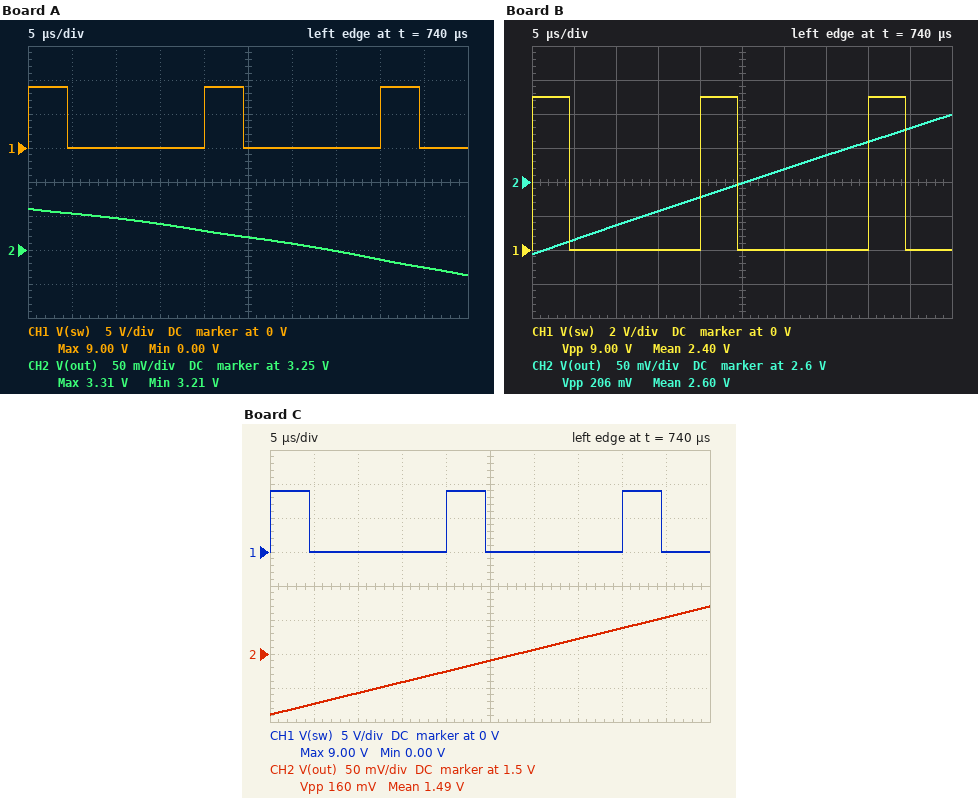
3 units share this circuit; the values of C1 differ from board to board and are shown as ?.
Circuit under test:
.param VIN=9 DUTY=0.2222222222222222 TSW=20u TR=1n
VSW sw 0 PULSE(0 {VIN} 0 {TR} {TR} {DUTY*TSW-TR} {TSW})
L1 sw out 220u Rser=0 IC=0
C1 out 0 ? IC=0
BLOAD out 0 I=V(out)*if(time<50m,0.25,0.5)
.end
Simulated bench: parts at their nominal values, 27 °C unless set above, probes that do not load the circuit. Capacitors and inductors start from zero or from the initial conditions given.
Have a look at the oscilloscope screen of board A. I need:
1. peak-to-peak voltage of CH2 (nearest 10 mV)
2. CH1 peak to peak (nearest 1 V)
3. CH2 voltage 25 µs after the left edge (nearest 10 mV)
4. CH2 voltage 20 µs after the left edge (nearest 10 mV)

100 mV
9 V
3.27 V
3.28 V
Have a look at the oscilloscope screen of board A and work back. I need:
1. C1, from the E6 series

220 µF
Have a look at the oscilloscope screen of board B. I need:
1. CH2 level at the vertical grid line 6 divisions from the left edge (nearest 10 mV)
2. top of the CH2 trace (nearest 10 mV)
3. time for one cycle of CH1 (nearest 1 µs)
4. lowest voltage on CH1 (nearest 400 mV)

2.62 V
2.70 V
20 µs
0 V
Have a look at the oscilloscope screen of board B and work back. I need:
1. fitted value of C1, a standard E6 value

680 µF
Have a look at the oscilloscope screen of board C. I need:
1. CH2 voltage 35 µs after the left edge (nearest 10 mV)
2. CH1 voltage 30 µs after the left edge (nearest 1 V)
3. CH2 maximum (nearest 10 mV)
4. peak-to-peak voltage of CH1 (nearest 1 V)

1.52 V
0 V
1.57 V
9 V
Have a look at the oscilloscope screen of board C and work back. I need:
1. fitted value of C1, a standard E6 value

1.5 mF
